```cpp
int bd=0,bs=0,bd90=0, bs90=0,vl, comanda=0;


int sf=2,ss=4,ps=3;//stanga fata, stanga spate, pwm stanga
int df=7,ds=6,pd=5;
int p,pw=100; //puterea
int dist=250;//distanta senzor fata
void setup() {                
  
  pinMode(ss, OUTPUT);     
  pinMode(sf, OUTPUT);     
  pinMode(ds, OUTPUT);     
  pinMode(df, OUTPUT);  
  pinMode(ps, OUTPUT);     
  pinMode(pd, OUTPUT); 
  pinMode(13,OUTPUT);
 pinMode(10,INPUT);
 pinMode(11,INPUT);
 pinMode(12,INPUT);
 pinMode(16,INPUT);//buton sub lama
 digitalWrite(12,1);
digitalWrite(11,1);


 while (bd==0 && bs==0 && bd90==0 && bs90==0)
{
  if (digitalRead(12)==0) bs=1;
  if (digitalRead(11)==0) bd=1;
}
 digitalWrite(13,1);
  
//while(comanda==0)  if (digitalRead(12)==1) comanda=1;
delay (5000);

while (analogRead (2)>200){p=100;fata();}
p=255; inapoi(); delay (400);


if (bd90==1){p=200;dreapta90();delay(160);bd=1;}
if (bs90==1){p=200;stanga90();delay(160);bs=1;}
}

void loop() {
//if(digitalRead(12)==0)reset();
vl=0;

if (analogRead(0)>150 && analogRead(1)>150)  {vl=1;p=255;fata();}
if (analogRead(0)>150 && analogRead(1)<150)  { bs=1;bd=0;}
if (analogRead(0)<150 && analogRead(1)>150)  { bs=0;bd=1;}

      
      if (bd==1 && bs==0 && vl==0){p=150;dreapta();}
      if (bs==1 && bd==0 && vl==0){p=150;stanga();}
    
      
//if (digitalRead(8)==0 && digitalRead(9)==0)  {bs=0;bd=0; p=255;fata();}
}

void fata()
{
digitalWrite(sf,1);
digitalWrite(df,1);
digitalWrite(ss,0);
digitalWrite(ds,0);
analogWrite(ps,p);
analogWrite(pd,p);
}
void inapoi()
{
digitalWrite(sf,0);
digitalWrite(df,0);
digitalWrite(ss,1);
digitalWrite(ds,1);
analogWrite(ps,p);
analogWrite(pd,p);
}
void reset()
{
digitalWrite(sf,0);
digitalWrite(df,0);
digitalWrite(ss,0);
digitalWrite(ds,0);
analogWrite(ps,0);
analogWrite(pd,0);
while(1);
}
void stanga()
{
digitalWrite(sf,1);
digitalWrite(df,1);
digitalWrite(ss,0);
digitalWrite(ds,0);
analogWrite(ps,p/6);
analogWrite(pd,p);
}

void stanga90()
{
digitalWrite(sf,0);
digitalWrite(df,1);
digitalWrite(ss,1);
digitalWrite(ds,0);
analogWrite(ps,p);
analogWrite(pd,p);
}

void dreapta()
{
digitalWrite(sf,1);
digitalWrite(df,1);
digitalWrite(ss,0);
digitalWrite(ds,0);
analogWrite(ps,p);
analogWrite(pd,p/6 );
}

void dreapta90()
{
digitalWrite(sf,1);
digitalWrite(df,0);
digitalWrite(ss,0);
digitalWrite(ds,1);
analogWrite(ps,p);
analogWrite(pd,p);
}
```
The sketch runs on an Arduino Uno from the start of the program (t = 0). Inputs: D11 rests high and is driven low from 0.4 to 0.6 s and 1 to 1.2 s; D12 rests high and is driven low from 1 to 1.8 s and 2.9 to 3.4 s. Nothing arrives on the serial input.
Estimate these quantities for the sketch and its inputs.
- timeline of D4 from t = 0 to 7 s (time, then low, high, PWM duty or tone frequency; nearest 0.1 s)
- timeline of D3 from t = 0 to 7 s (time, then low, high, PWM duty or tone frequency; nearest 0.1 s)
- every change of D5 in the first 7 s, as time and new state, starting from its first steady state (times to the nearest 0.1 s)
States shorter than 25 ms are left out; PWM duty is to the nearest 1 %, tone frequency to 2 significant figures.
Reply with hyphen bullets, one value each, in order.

- 0 s low; 5.4 s high; 5.8 s low
- 0 s low; 5.4 s high; 5.8 s PWM 59 %
- 0 s low; 5.4 s high; 5.8 s PWM 10 %
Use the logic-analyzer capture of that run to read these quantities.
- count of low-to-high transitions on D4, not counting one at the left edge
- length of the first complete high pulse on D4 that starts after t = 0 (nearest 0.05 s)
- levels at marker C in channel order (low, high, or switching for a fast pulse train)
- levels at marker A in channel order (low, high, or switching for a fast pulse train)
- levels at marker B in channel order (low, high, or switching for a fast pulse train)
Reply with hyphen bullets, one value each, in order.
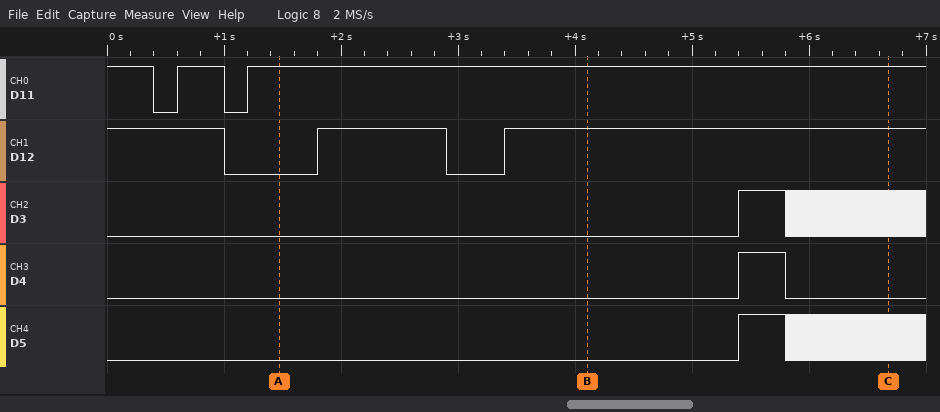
- 1
- 0.40 s
- D11 high, D12 high, D3 switching, D4 low, D5 switching
- D11 high, D12 low, D3 low, D4 low, D5 low
- D11 high, D12 high, D3 low, D4 low, D5 low
